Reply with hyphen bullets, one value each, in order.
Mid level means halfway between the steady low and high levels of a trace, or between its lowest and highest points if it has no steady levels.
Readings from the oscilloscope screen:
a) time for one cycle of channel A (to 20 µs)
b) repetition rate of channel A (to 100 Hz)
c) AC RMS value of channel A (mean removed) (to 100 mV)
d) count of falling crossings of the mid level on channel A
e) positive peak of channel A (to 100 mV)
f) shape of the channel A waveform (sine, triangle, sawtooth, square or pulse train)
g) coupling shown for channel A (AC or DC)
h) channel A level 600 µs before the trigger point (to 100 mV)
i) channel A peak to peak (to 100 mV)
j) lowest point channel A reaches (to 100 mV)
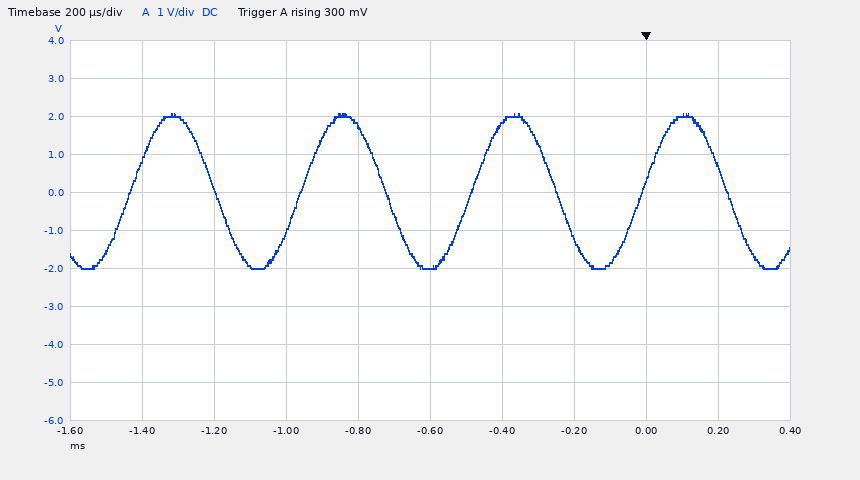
- 480 µs
- 2.1 kHz
- 1.4 V
- 4
- 2.1 V
- sine
- DC
- -2.0 V
- 4.1 V
- -2.0 V
